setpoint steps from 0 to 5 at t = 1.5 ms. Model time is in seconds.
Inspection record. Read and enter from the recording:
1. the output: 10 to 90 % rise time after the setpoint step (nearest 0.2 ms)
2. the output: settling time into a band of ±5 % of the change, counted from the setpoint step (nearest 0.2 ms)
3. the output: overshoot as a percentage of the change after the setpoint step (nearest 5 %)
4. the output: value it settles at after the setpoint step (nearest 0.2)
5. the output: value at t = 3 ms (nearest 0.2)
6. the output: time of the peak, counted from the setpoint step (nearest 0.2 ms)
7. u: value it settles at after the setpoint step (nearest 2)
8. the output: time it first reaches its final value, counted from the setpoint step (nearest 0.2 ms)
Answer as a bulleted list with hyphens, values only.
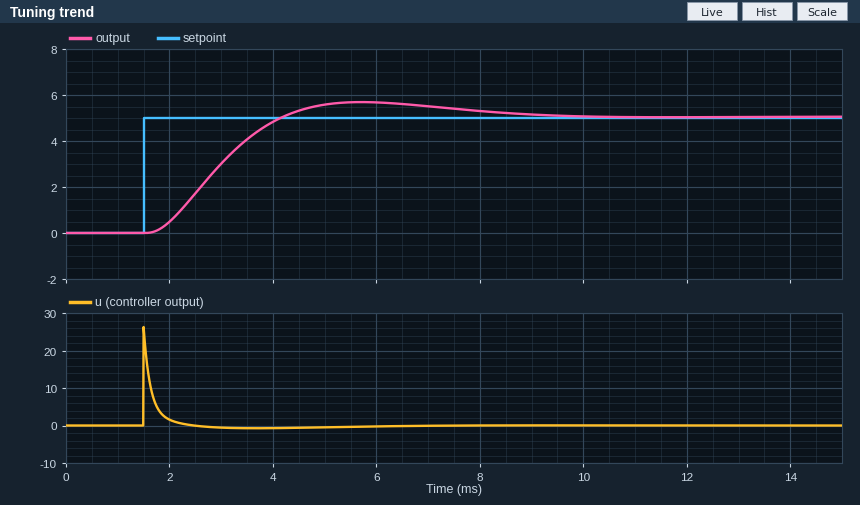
- 1.8 ms
- 6.6 ms
- 15 %
- 5.0
- 3.0
- 4.2 ms
- 0
- 2.6 ms
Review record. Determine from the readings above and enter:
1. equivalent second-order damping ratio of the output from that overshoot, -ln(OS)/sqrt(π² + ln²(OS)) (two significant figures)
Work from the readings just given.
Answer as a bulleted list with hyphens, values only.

- 0.52
